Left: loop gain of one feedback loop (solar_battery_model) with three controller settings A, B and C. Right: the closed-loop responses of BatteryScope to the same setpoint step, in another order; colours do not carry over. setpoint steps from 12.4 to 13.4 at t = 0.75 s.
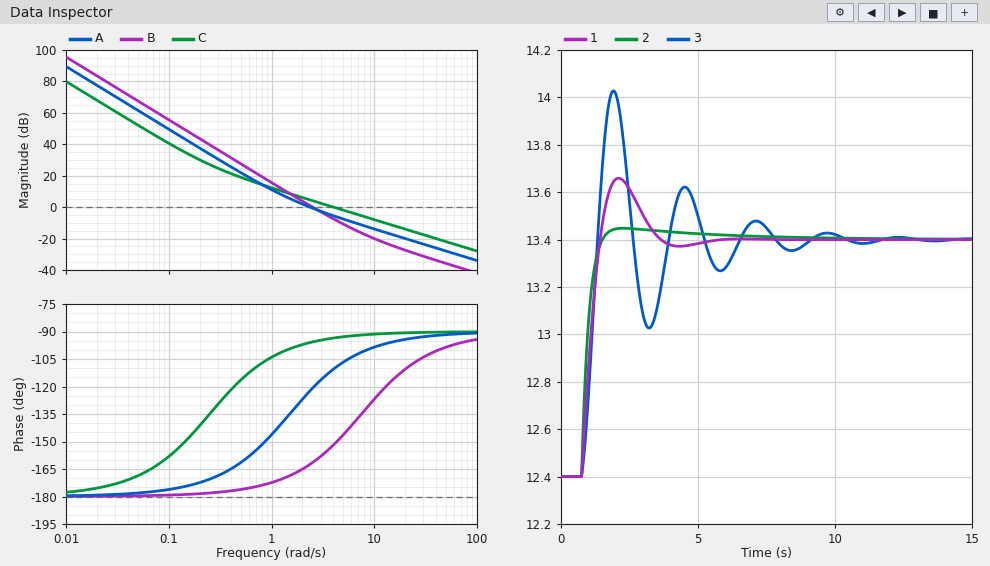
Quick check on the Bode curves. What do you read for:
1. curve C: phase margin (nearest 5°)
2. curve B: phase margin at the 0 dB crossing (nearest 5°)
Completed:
85°
20°
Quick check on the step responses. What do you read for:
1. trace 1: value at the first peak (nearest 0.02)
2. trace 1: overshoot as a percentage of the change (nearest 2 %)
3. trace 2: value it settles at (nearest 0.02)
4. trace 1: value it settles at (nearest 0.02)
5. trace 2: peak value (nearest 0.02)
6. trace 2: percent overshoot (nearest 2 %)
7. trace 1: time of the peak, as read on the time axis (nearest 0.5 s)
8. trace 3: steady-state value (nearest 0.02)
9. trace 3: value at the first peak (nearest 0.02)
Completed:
13.66
26 %
13.40
13.40
13.44
4 %
2.0 s
13.40
14.02
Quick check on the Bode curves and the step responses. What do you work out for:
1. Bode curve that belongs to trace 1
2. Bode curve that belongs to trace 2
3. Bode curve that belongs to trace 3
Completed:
A
C
B
